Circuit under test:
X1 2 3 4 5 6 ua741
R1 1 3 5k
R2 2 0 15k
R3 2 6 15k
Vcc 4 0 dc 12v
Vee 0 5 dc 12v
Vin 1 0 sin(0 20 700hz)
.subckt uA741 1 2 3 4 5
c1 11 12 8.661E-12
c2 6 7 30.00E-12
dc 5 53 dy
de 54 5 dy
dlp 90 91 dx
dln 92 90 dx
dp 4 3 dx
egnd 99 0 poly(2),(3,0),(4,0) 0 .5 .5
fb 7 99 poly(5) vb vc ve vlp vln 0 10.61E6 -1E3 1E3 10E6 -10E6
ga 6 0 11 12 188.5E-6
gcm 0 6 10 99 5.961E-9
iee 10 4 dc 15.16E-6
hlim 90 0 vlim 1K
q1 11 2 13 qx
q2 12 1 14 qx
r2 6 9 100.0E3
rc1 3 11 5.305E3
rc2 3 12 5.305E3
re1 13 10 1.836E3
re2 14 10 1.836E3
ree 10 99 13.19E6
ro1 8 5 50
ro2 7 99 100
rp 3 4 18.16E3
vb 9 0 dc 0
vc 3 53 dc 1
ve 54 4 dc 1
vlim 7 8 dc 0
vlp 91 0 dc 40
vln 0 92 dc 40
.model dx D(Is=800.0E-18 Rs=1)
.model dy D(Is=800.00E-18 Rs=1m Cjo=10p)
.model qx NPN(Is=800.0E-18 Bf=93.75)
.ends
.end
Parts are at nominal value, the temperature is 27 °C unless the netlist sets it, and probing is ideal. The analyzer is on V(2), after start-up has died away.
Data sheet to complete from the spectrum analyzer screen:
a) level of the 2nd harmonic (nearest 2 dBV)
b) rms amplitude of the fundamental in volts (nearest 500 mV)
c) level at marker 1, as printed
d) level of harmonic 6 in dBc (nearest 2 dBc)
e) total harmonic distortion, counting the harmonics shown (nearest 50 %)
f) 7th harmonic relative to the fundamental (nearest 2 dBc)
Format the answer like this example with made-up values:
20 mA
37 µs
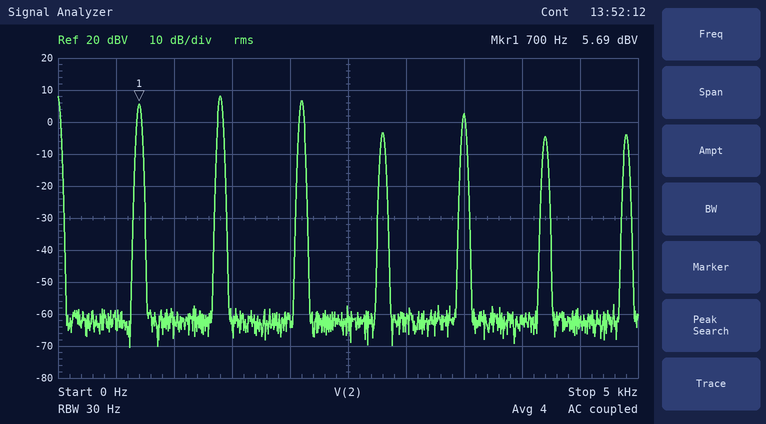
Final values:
8 dBV
2.0 V
5.69 dBV
-10 dBc
200 %
-10 dBc
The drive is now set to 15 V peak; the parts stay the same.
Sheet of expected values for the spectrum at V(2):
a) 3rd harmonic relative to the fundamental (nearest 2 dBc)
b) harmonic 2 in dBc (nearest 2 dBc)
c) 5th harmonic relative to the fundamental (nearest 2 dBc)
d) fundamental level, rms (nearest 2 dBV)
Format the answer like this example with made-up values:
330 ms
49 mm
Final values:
0 dBc
-2 dBc
-8 dBc
10 dBV
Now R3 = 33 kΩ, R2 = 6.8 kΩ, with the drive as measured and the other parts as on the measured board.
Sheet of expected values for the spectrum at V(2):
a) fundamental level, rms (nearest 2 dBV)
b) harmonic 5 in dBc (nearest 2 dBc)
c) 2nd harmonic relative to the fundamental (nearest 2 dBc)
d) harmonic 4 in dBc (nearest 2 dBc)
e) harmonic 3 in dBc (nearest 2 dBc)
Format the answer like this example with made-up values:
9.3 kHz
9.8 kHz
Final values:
-8 dBV
4 dBc
6 dBc
-6 dBc
6 dBc
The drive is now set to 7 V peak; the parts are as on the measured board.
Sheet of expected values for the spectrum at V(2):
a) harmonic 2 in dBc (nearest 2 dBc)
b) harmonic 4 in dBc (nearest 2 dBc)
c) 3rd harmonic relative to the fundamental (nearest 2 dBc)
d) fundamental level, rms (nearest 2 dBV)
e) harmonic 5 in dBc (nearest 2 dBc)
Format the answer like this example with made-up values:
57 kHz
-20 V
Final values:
-52 dBc
-52 dBc
-10 dBc
14 dBV
-14 dBc
